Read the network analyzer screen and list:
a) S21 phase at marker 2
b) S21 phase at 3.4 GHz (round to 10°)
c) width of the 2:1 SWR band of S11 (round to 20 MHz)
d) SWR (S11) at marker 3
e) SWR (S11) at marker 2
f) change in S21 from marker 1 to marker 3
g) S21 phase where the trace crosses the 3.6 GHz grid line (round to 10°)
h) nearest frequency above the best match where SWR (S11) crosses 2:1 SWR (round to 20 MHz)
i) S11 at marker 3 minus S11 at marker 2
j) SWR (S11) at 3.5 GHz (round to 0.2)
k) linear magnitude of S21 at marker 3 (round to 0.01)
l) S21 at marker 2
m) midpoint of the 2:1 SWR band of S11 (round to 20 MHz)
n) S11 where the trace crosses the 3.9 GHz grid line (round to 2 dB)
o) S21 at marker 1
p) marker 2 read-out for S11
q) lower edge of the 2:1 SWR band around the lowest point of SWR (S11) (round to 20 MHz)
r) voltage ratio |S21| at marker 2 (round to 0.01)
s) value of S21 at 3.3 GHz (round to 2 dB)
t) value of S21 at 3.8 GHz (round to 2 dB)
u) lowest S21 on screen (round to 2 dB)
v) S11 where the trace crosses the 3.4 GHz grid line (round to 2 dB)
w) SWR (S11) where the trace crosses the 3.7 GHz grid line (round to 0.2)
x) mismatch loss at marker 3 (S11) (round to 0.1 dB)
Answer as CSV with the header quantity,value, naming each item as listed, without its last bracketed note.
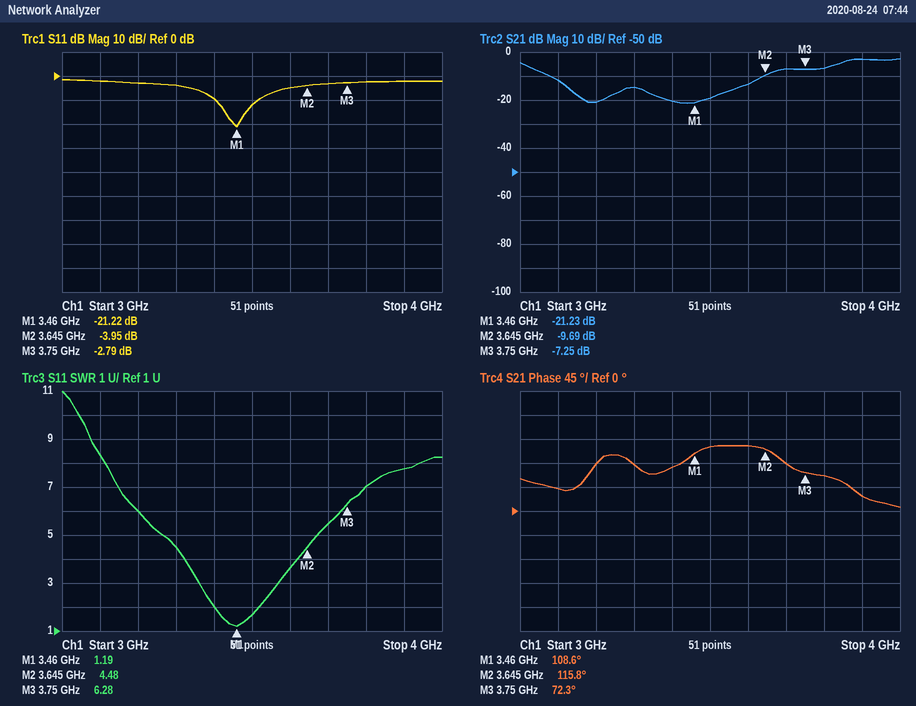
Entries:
quantity,value
S21 phase at marker 2,115.8°
S21 phase at 3.4 GHz,80°
width of the 2:1 SWR band of S11,120 MHz
SWR (S11) at marker 3,6.28
SWR (S11) at marker 2,4.48
change in S21 from marker 1 to marker 3,13.98 dB
S21 phase where the trace crosses the 3.6 GHz grid line,120°
nearest frequency above the best match where SWR (S11) crosses 2:1 SWR,3.52 GHz
S11 at marker 3 minus S11 at marker 2,1.16 dB
SWR (S11) at 3.5 GHz,1.6
linear magnitude of S21 at marker 3,0.43
S21 at marker 2,-9.69 dB
midpoint of the 2:1 SWR band of S11,3.46 GHz
S11 where the trace crosses the 3.9 GHz grid line,-2 dB
S21 at marker 1,-21.23 dB
marker 2 read-out for S11,-3.95 dB
lower edge of the 2:1 SWR band around the lowest point of SWR (S11),3.40 GHz
voltage ratio |S21| at marker 2,0.33
value of S21 at 3.3 GHz,-14 dB
value of S21 at 3.8 GHz,-6 dB
lowest S21 on screen,-22 dB
S11 where the trace crosses the 3.4 GHz grid line,-10 dB
SWR (S11) where the trace crosses the 3.7 GHz grid line,5.4
mismatch loss at marker 3 (S11),3.2 dB
